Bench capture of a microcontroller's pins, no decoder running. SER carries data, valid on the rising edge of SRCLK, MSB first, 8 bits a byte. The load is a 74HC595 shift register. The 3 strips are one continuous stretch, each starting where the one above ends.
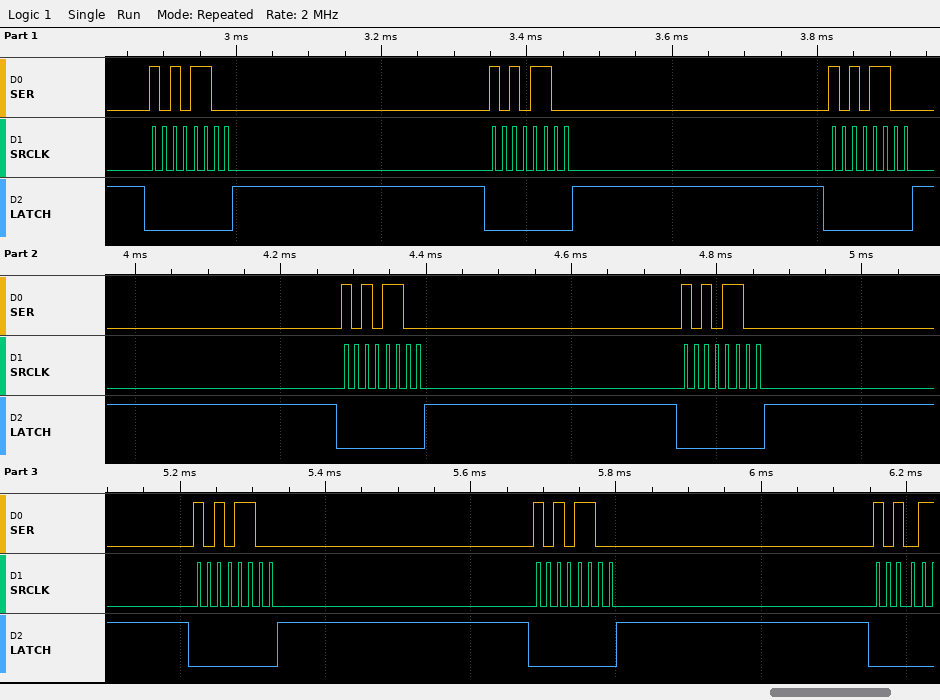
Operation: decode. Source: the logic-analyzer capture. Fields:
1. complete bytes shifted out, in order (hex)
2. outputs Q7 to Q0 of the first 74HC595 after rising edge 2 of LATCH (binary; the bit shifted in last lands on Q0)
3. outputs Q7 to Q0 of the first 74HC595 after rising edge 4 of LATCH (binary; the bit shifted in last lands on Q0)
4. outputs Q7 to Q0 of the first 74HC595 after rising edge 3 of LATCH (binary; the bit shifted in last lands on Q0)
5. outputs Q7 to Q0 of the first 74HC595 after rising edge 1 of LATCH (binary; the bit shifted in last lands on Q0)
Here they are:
AC AC AC AC AC AC AC
10101100
10101100
10101100
10101100
